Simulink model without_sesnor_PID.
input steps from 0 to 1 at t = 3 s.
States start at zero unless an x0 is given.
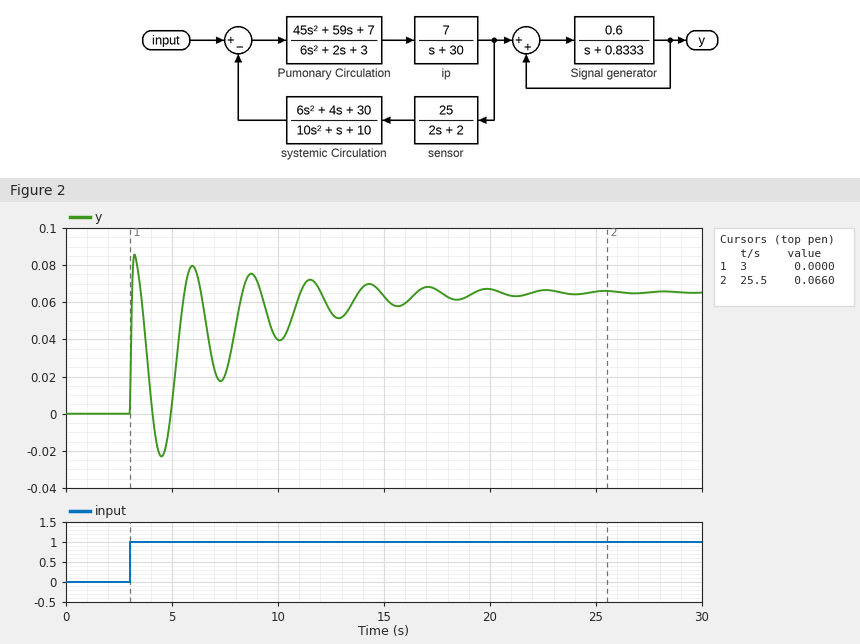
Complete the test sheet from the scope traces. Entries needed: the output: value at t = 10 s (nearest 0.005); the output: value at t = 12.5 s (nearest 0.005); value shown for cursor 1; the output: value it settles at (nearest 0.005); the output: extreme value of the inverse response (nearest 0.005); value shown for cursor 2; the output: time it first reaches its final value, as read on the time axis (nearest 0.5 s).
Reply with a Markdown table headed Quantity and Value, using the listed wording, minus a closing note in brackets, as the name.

| Quantity | Value |
|---|---|
| the output: value at t = 10 s | 0.040 |
| the output: value at t = 12.5 s | 0.055 |
| value shown for cursor 1 | 0.0000 |
| the output: value it settles at | 0.065 |
| the output: extreme value of the inverse response | -0.025 |
| value shown for cursor 2 | 0.0660 |
| the output: time it first reaches its final value, as read on the time axis | 3.0 s |
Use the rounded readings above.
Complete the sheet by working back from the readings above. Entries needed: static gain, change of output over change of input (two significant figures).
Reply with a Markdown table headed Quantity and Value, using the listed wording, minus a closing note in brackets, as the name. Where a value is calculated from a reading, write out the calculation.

| Quantity | Value |
|---|---|
| static gain, change of output over change of input | (0.065 - 0) / (1 - 0) = 0.065 |
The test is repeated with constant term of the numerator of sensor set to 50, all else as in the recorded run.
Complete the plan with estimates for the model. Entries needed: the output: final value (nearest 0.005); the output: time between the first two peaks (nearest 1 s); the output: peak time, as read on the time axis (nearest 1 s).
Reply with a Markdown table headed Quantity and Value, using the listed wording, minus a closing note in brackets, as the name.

| Quantity | Value |
|---|---|
| the output: final value | 0.035 |
| the output: time between the first two peaks | 3 s |
| the output: peak time, as read on the time axis | 3 s |
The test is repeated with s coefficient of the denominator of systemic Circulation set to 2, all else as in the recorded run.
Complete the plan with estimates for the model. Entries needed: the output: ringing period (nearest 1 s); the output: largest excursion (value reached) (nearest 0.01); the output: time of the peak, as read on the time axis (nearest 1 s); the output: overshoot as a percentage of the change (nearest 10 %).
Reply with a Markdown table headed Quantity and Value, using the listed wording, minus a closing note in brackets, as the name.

| Quantity | Value |
|---|---|
| the output: ringing period | 3 s |
| the output: largest excursion (value reached) | 0.09 |
| the output: time of the peak, as read on the time axis | 3 s |
| the output: overshoot as a percentage of the change | 30 % |
